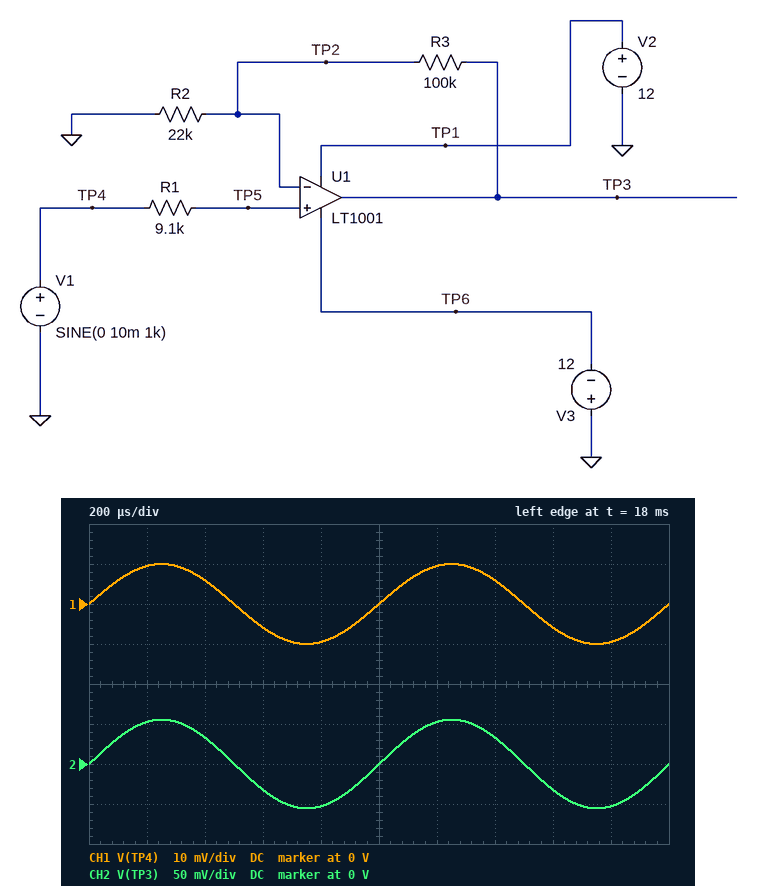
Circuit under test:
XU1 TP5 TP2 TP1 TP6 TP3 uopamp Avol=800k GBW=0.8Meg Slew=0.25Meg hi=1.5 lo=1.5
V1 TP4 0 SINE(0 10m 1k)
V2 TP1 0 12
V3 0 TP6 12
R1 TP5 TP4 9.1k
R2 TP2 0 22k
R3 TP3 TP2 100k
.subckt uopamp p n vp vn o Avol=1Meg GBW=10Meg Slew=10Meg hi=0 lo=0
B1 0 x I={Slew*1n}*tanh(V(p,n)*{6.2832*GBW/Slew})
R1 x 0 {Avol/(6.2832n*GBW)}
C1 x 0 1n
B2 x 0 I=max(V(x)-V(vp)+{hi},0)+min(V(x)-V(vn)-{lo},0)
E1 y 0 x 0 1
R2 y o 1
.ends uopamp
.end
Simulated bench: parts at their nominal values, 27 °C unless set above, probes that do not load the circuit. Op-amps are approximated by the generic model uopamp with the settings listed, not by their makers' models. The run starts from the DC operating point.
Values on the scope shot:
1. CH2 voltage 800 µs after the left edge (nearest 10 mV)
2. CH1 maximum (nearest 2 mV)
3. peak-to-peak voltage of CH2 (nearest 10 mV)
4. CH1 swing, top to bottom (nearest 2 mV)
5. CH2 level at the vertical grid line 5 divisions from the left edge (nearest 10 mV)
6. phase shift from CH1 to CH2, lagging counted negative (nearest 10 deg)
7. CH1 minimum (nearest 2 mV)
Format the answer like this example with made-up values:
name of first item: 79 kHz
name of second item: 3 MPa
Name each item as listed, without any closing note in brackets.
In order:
CH2 voltage 800 µs after the left edge: -50 mV
CH1 maximum: 10 mV
peak-to-peak voltage of CH2: 110 mV
CH1 swing, top to bottom: 20 mV
CH2 level at the vertical grid line 5 divisions from the left edge: 0 V
phase shift from CH1 to CH2, lagging counted negative: 0 deg
CH1 minimum: -10 mV
